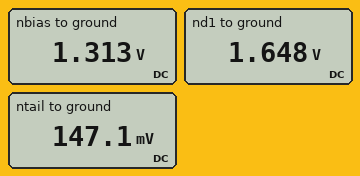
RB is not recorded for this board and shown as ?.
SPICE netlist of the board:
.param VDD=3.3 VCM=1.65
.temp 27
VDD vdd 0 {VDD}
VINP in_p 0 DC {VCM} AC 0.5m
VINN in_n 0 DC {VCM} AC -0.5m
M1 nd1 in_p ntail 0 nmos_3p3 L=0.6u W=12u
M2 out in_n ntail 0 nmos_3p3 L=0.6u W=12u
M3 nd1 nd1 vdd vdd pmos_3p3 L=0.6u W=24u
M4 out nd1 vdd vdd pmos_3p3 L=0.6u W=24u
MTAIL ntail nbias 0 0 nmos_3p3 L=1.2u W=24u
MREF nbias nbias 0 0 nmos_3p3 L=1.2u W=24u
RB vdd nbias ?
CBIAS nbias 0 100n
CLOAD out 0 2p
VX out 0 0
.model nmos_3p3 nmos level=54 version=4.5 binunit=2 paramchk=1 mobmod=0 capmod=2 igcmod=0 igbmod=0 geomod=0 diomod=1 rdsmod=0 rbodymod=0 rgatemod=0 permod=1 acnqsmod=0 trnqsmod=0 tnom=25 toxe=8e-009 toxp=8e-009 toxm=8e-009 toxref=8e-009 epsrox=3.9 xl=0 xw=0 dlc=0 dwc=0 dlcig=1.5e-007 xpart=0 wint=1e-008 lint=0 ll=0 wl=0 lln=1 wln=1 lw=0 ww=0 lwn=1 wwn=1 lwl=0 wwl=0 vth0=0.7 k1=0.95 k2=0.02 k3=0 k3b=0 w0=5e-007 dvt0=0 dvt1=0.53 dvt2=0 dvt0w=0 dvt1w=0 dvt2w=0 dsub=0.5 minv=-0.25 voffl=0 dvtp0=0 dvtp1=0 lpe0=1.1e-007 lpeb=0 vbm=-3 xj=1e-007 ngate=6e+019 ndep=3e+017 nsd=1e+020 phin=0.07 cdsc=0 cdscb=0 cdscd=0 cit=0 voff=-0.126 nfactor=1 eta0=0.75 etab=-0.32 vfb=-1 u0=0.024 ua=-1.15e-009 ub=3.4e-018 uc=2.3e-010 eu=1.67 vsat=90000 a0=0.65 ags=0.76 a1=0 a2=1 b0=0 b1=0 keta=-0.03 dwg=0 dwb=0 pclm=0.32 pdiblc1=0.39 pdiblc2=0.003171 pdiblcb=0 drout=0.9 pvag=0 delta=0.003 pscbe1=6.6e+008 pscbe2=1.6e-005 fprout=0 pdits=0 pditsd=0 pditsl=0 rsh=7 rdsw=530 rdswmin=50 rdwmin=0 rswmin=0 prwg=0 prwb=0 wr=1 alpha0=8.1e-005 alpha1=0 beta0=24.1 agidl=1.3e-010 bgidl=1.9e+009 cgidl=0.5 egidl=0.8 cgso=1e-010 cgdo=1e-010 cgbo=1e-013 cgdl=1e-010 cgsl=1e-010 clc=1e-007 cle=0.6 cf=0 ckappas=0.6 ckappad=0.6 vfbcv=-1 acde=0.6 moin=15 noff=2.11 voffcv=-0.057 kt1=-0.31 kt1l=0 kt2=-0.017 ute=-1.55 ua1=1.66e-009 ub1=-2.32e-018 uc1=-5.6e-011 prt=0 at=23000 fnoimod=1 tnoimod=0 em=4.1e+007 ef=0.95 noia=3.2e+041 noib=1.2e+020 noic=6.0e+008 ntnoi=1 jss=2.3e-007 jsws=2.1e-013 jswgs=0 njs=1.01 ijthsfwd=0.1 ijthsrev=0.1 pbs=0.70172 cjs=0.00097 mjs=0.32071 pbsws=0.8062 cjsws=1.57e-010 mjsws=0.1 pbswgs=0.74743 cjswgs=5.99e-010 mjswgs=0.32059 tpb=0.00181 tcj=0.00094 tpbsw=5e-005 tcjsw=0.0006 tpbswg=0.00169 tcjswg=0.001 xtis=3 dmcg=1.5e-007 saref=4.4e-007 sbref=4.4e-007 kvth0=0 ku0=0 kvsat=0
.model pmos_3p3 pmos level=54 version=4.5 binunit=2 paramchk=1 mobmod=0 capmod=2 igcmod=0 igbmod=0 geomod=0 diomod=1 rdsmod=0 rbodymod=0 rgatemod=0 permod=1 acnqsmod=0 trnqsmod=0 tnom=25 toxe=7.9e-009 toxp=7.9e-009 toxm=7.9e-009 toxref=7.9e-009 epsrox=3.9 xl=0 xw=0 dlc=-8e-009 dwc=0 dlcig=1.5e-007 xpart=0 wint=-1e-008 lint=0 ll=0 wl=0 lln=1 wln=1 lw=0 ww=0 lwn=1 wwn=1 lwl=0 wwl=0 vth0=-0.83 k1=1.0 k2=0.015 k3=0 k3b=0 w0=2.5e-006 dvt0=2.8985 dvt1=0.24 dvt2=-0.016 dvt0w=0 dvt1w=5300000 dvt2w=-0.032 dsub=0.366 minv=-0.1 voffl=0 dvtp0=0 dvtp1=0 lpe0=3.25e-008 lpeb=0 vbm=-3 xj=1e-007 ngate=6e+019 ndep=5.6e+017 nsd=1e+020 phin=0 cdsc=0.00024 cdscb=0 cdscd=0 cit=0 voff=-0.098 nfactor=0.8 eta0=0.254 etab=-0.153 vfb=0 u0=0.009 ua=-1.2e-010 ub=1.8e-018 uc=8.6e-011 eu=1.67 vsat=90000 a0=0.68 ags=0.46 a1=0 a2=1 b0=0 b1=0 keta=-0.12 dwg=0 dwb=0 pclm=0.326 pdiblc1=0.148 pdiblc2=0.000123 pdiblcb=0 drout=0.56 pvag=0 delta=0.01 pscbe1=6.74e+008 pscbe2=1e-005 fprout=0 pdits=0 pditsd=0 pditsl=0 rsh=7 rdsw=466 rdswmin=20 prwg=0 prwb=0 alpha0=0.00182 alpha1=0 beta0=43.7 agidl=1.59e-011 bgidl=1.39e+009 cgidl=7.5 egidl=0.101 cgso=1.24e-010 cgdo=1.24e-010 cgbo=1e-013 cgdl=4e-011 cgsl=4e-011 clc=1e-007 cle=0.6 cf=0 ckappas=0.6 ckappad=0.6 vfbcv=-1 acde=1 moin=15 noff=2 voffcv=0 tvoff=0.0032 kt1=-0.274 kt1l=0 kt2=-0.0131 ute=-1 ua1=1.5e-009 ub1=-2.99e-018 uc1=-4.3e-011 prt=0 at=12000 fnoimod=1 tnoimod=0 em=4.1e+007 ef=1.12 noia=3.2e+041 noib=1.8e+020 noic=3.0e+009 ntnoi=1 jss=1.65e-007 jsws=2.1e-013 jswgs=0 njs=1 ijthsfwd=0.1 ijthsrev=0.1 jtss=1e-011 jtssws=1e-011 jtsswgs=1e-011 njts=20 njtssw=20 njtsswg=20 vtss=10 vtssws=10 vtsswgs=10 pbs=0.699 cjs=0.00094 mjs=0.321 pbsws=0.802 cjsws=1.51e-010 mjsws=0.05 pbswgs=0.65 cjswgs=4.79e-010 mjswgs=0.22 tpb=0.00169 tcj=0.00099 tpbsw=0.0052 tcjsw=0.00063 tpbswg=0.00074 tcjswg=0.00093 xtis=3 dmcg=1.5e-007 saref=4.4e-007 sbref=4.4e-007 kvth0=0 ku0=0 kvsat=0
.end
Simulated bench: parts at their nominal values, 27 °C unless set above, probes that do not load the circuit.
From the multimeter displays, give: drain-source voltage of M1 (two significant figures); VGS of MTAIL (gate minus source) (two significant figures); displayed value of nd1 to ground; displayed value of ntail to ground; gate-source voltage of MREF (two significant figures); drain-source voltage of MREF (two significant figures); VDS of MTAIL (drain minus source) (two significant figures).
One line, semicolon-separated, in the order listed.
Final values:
1.5 V; 1.3 V; 1.648 V; 147.1 mV; 1.3 V; 1.3 V; 150 mV
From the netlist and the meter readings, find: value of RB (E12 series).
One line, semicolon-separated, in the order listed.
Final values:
6.8 kΩ
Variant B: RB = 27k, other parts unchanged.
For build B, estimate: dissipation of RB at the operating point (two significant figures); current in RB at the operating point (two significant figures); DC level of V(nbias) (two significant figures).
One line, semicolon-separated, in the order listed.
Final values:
190 µW; 84 µA; 1.0 V
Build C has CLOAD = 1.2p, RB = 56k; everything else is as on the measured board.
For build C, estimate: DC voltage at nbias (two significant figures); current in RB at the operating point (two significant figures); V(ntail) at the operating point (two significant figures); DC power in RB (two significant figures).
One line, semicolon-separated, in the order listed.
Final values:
940 mV; 42 µA; 190 mV; 100 µW
